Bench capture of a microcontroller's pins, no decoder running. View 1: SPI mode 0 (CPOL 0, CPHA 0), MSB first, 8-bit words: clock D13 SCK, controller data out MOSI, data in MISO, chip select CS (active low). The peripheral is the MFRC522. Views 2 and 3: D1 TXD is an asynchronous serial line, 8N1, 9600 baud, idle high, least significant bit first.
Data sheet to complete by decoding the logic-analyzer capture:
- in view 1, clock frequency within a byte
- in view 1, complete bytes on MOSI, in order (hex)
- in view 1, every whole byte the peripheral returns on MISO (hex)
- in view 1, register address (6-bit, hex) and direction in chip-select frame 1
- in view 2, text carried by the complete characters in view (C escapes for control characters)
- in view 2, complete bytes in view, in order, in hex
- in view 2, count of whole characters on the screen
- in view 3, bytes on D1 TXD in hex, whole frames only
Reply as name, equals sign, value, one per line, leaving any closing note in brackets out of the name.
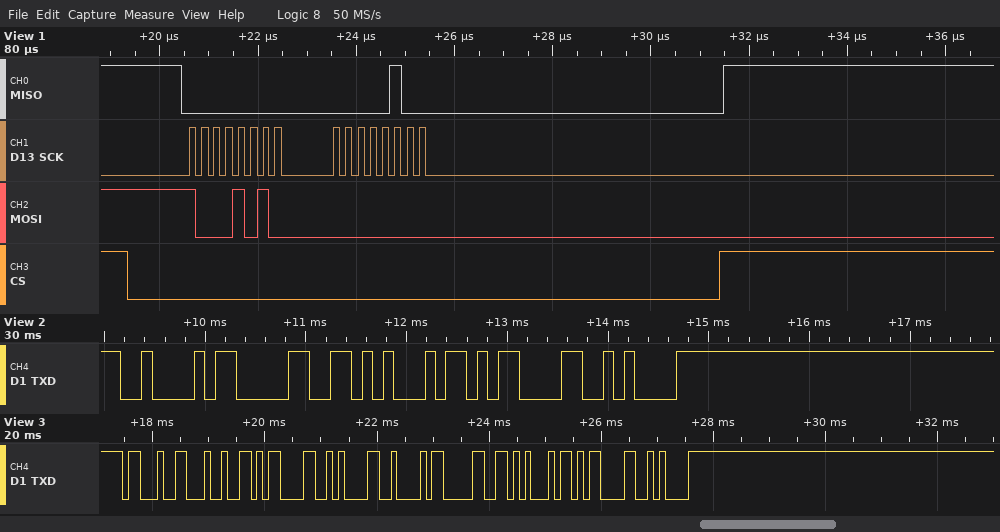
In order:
in view 1, clock frequency within a byte = 4 MHz
in view 1, complete bytes on MOSI, in order = 0x8A 0x00
in view 1, every whole byte the peripheral returns on MISO = 0x00 0x04
in view 1, register address (6-bit, hex) and direction in chip-select frame 1 = 0x05 read
in view 2, text carried by the complete characters in view = "B0E\r\n"
in view 2, complete bytes in view, in order, in hex = 42 30 45 0D 0A
in view 2, count of whole characters on the screen = 5
in view 3, bytes on D1 TXD in hex, whole frames only = 23 24 0D 0A 42 30 45 0D 0A
